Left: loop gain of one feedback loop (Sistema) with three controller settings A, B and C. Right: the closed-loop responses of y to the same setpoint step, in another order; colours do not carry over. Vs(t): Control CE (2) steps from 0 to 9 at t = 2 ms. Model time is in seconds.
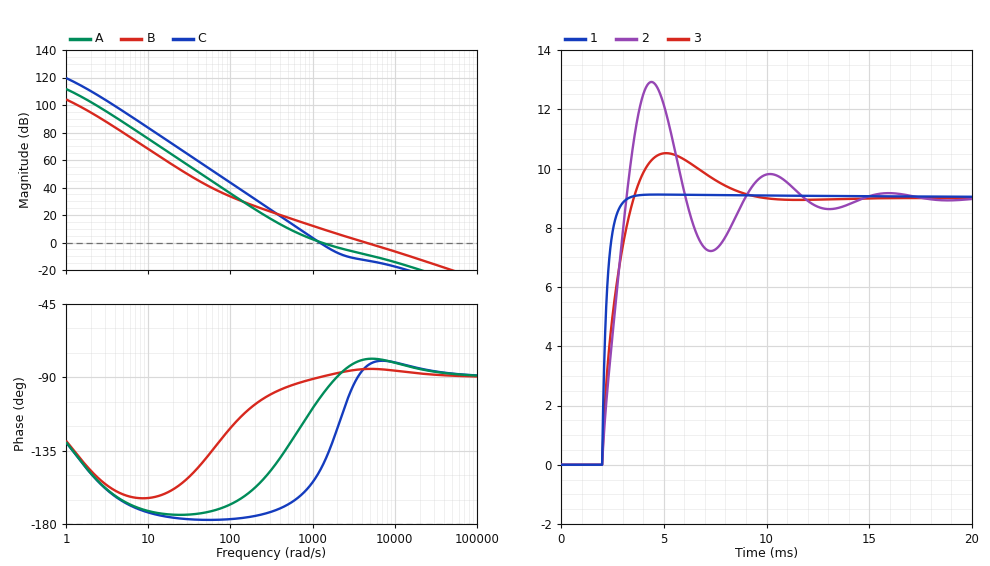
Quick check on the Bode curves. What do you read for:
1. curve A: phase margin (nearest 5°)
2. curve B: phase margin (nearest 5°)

80°
95°
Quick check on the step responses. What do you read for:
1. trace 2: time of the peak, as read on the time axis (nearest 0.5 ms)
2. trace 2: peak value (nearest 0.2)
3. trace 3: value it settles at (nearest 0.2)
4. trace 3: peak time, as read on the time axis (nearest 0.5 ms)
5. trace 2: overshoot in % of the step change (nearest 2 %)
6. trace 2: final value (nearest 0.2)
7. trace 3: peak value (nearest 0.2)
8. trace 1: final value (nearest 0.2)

4.5 ms
13.0
9.0
5.0 ms
44 %
9.0
10.6
9.0
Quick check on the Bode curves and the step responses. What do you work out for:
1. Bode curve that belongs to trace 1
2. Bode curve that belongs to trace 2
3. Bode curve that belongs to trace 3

B
C
A
